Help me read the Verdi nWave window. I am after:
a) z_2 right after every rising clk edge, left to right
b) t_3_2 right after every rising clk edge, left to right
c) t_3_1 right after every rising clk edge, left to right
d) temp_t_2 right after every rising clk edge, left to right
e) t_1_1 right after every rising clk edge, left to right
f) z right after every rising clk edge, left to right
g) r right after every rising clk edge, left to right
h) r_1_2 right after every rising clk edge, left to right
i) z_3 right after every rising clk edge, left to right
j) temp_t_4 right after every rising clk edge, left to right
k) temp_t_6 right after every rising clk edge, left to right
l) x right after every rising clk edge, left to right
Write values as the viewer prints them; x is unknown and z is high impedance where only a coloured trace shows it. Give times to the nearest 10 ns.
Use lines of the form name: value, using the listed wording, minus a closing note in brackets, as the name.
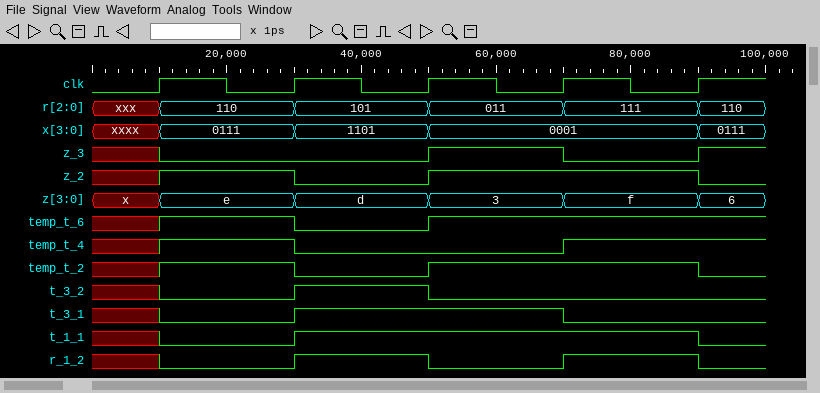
z_2 right after every rising clk edge, left to right: 1 0 1 1 0
t_3_2 right after every rising clk edge, left to right: 0 1 0 0 0
t_3_1 right after every rising clk edge, left to right: 0 1 1 0 0
temp_t_2 right after every rising clk edge, left to right: 1 0 1 1 0
t_1_1 right after every rising clk edge, left to right: 0 1 1 1 0
z right after every rising clk edge, left to right: e, d, 3, f, 6
r right after every rising clk edge, left to right: 110, 101, 011, 111, 110
r_1_2 right after every rising clk edge, left to right: 0 1 0 1 0
z_3 right after every rising clk edge, left to right: 0 0 1 0 1
temp_t_4 right after every rising clk edge, left to right: 1 0 0 1 1
temp_t_6 right after every rising clk edge, left to right: 1 0 1 1 1
x right after every rising clk edge, left to right: 0111, 1101, 0001, 0001, 0111
